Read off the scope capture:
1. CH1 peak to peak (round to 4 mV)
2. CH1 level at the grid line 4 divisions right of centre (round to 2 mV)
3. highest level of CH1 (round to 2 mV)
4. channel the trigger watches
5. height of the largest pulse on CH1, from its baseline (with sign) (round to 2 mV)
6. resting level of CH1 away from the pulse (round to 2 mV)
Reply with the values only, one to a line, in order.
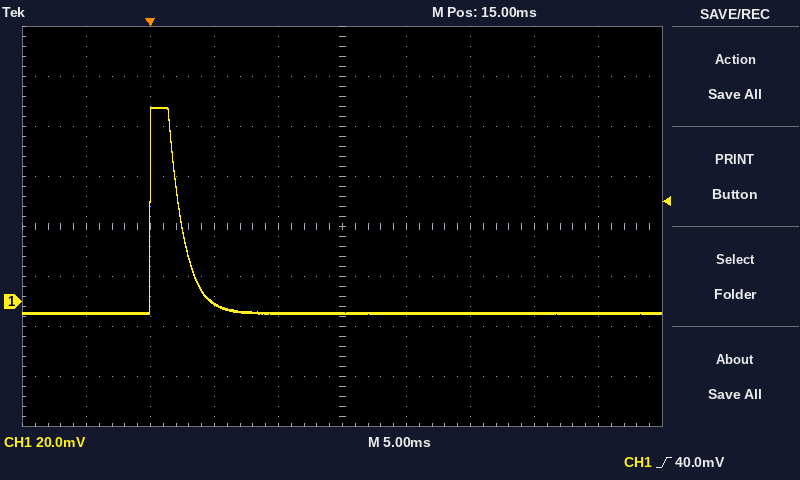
84 mV
-4 mV
78 mV
CH1
+82 mV
-4 mV
